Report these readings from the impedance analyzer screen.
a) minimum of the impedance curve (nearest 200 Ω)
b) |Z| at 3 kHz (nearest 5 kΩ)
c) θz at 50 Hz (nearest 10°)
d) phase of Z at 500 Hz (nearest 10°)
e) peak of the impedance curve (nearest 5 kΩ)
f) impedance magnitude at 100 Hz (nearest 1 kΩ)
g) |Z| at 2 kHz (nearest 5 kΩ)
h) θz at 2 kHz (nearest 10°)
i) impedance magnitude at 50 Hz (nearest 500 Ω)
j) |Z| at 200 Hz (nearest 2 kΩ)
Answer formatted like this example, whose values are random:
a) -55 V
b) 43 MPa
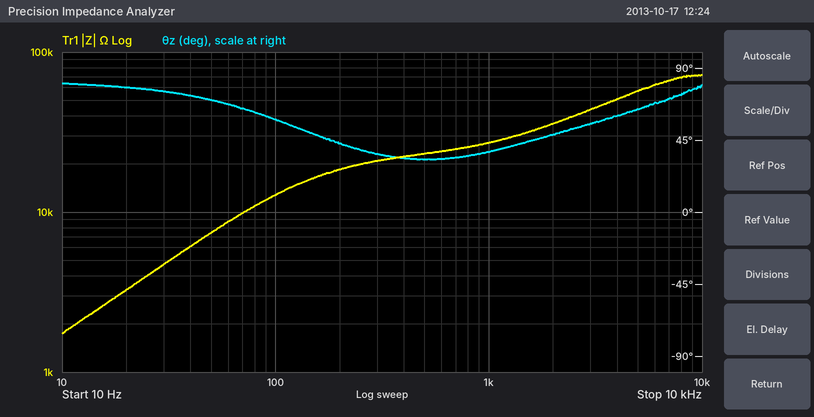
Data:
a) 1.8 kΩ
b) 45 kΩ
c) 70°
d) 30°
e) 70 kΩ
f) 13 kΩ
g) 35 kΩ
h) 50°
i) 7.5 kΩ
j) 18 kΩ
